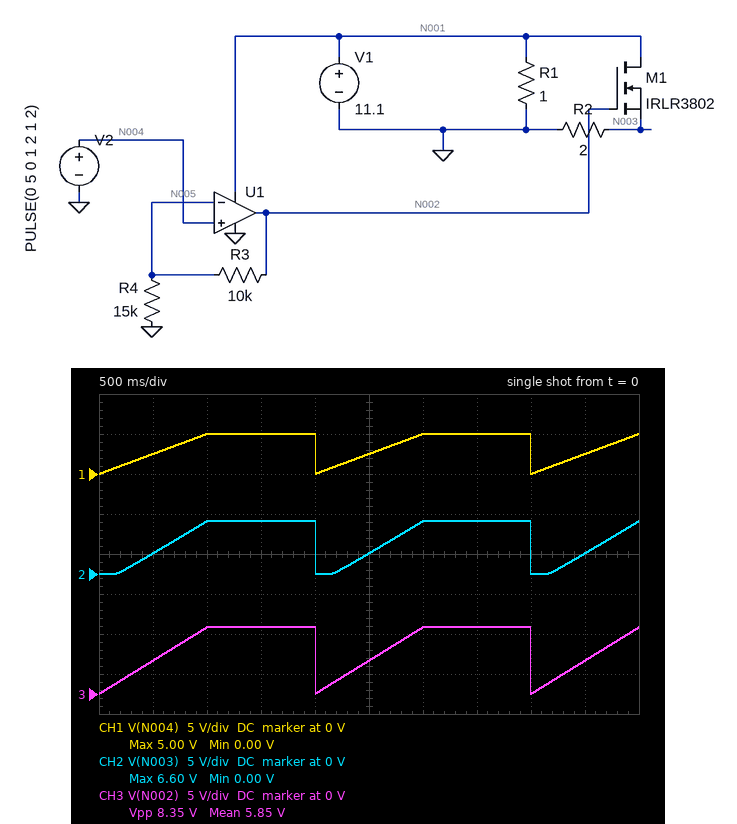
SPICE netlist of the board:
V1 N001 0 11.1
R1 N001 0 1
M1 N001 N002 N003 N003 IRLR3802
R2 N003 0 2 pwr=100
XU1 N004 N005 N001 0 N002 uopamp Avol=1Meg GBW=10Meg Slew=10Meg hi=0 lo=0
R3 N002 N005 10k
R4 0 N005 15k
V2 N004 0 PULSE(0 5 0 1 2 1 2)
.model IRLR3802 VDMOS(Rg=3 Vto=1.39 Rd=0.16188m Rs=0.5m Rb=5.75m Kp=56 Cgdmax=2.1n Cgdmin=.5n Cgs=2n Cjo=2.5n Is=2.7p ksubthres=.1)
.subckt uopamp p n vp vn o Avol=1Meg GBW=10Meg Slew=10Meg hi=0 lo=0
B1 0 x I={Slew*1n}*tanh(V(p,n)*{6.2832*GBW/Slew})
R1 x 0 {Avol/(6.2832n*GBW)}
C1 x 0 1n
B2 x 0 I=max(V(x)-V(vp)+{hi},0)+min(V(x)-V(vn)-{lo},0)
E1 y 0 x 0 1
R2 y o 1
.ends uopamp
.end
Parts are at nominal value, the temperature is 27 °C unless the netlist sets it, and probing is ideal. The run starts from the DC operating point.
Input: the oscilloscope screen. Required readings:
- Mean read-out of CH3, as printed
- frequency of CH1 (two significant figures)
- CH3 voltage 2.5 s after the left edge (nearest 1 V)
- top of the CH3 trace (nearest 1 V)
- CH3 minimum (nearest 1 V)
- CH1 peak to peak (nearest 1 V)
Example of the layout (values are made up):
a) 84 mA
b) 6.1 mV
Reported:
a) 5.85 V
b) 500 mHz
c) 4 V
d) 8 V
e) 0 V
f) 5 V
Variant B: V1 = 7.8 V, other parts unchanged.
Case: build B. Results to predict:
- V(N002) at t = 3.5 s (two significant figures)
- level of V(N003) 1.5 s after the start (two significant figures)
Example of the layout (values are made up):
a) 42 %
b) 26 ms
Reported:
a) 7.8 V
b) 6.1 V
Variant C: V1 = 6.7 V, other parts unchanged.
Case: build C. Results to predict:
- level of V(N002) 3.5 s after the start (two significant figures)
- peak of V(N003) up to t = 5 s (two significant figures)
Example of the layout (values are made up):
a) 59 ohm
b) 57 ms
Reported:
a) 6.7 V
b) 5.0 V
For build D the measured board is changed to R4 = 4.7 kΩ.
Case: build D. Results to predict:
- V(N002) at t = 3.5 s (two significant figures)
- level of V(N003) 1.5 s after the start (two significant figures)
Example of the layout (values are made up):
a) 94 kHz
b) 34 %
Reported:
a) 11 V
b) 9.3 V
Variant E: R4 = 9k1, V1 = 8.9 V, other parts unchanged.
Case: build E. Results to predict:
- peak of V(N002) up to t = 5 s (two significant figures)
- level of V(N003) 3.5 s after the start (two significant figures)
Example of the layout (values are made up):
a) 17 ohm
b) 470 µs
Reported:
a) 8.9 V
b) 7.2 V
